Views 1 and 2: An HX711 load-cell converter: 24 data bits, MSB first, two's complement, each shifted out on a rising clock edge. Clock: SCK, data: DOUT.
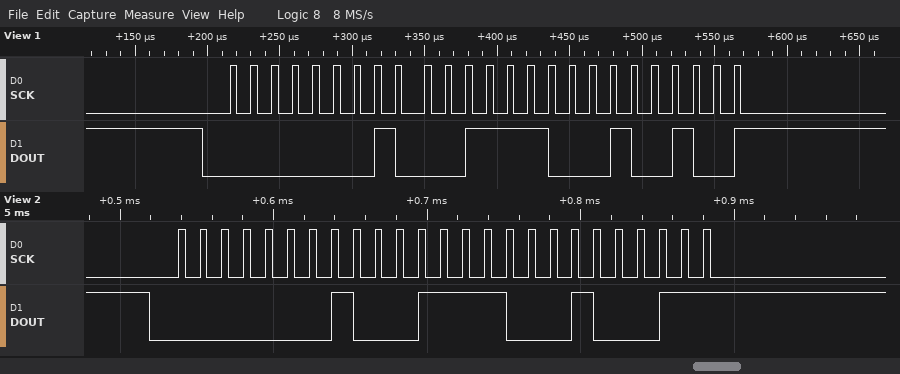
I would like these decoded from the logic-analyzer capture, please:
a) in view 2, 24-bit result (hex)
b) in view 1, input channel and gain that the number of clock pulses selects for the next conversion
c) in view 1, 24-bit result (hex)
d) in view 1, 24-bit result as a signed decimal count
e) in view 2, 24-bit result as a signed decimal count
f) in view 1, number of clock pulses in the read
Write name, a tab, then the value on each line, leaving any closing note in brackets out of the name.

in view 2, 24-bit result	0x011E23
in view 1, input channel and gain that the number of clock pulses selects for the next conversion	channel A, gain 128
in view 1, 24-bit result	0x011E24
in view 1, 24-bit result as a signed decimal count	73252
in view 2, 24-bit result as a signed decimal count	73251
in view 1, number of clock pulses in the read	25
